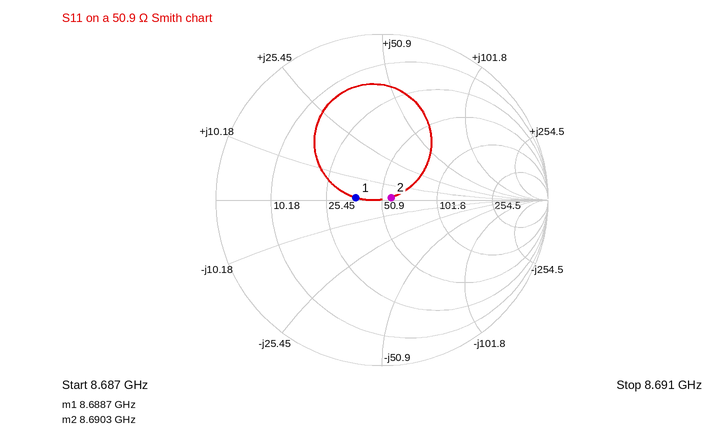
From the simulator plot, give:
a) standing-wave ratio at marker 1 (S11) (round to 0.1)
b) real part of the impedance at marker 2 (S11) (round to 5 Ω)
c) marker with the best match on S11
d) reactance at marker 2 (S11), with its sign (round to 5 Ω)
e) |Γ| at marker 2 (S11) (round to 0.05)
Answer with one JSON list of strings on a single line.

["1.4", "55 Ω", "marker 2", "0 Ω", "0.05"]
